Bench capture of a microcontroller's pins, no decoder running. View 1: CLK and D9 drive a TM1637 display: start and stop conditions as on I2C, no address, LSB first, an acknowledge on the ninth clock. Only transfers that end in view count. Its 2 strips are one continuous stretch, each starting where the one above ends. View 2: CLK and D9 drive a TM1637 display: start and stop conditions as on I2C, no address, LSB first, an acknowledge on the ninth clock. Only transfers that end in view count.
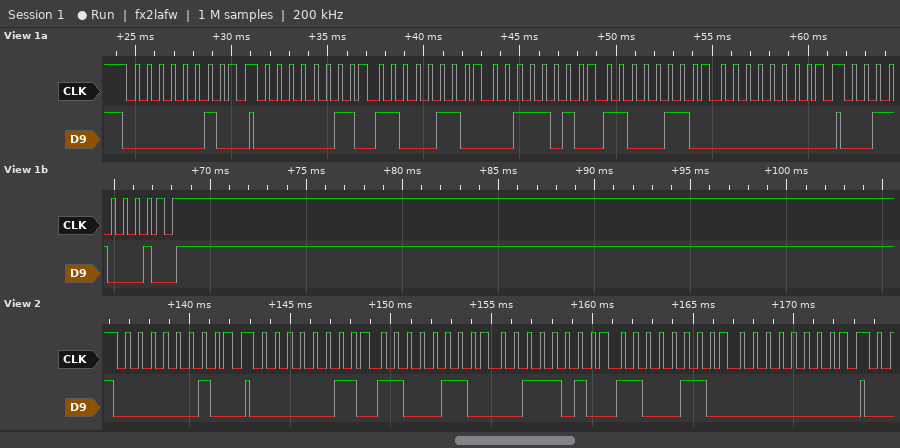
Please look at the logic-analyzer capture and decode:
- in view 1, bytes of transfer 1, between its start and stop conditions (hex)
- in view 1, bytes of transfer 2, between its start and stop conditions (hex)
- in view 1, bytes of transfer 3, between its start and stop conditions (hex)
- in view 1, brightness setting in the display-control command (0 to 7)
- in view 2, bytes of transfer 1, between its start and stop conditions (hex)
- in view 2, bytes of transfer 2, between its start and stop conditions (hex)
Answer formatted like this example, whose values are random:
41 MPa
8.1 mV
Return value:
40
C0 63 5C 63 00
8C
4
40
C0 63 5C 63 00
